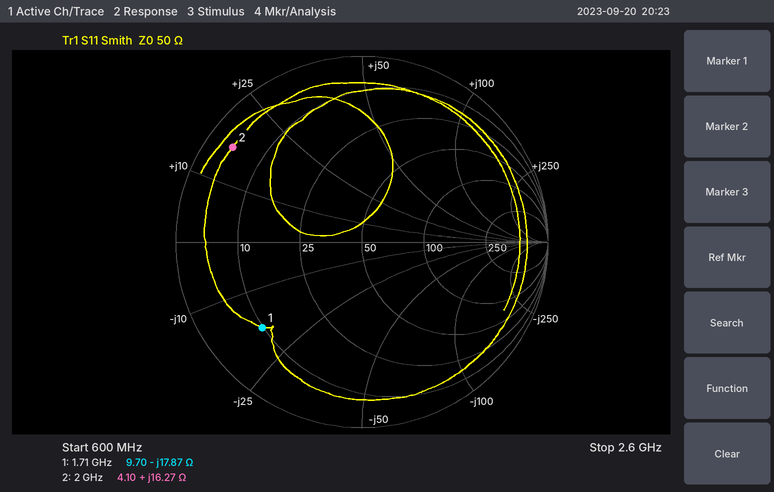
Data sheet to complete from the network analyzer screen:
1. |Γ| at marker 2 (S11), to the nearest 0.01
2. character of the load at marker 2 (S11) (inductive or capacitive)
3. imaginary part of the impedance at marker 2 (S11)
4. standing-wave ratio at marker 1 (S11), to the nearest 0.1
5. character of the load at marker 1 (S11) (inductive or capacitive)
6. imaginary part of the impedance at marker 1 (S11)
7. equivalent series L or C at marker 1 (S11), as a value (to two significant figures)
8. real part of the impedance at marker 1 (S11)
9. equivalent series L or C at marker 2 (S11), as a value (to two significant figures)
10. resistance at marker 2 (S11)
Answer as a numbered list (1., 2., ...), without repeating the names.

1. 0.86
2. inductive
3. +16.27 Ω
4. 5.8
5. capacitive
6. -17.87 Ω
7. 5.2 pF
8. 9.70 Ω
9. 1.3 nH
10. 4.10 Ω
